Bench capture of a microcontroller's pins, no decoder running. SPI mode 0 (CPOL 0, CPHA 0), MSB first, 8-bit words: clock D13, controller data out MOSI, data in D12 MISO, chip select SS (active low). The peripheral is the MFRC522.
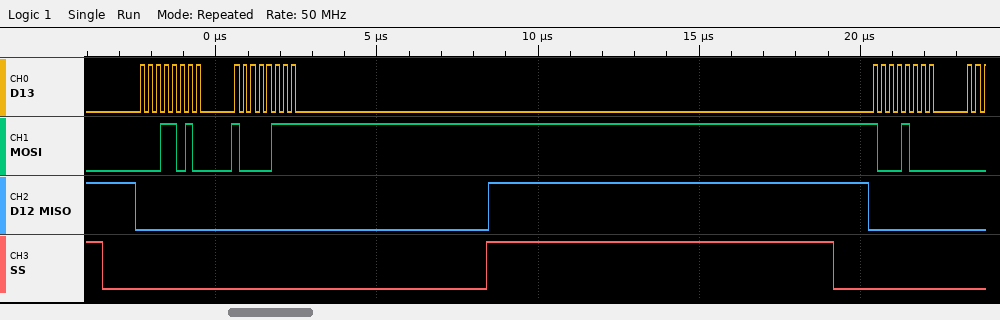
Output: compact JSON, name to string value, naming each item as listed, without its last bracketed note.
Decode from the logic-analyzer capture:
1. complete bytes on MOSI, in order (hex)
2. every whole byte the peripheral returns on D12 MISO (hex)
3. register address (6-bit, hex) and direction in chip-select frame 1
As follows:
{"complete bytes on MOSI, in order": "0x1A 0x87 0x88", "every whole byte the peripheral returns on D12 MISO": "0x00 0x00 0x00", "register address (6-bit, hex) and direction in chip-select frame 1": "0x0D write"}
